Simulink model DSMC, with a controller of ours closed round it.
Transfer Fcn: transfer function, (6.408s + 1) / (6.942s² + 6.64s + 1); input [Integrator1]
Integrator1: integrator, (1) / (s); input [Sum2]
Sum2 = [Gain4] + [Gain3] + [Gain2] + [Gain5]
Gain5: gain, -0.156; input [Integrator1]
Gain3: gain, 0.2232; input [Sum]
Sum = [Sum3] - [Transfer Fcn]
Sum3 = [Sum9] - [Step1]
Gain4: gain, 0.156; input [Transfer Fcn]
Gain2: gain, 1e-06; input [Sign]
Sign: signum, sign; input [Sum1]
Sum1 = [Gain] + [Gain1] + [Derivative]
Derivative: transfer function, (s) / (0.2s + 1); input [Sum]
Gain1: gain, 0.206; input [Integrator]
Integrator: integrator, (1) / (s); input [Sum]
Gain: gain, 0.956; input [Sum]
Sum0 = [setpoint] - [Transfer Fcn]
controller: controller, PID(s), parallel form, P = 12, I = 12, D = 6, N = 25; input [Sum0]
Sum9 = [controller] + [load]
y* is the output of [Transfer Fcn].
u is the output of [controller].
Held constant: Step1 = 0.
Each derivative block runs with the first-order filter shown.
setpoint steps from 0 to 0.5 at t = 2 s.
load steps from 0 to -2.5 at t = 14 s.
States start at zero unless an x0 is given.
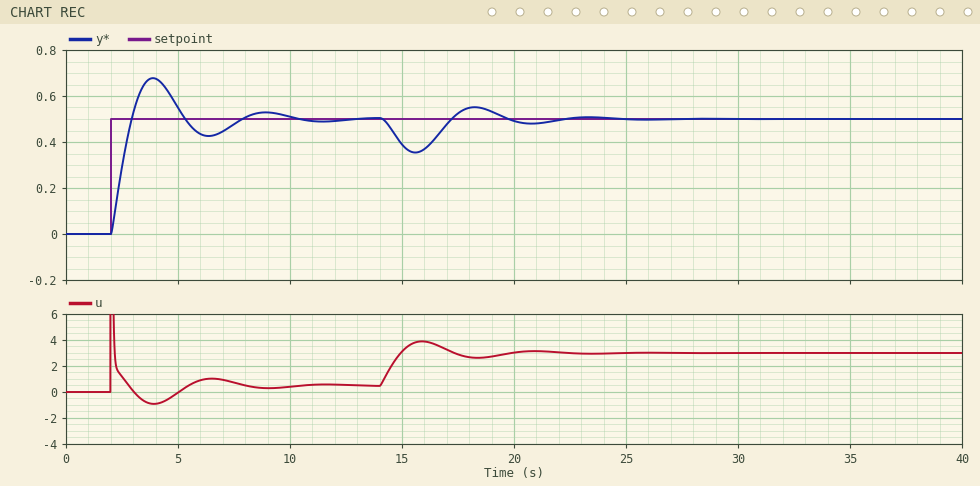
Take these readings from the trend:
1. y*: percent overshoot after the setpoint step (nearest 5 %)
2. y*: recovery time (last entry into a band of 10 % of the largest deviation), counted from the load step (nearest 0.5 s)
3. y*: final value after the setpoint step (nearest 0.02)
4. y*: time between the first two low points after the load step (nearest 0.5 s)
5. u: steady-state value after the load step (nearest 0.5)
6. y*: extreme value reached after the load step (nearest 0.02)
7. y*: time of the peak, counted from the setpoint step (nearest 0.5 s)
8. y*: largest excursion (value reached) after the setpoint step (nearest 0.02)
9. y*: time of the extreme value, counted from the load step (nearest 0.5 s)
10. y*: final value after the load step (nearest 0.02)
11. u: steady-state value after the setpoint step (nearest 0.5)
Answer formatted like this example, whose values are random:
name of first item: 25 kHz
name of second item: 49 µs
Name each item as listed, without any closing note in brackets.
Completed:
y*: percent overshoot after the setpoint step: 35 %
y*: recovery time (last entry into a band of 10 % of the largest deviation), counted from the load step: 7.5 s
y*: final value after the setpoint step: 0.50
y*: time between the first two low points after the load step: 5.0 s
u: steady-state value after the load step: 3.0
y*: extreme value reached after the load step: 0.36
y*: time of the peak, counted from the setpoint step: 2.0 s
y*: largest excursion (value reached) after the setpoint step: 0.68
y*: time of the extreme value, counted from the load step: 1.5 s
y*: final value after the load step: 0.50
u: steady-state value after the setpoint step: 0.5
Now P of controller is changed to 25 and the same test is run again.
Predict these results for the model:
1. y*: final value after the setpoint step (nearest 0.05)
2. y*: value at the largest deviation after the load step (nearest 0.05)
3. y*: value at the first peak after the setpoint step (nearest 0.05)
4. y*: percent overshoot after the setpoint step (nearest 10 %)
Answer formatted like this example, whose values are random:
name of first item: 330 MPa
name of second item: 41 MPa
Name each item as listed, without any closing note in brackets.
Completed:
y*: final value after the setpoint step: 0.50
y*: value at the largest deviation after the load step: 0.40
y*: value at the first peak after the setpoint step: 0.65
y*: percent overshoot after the setpoint step: 30 %
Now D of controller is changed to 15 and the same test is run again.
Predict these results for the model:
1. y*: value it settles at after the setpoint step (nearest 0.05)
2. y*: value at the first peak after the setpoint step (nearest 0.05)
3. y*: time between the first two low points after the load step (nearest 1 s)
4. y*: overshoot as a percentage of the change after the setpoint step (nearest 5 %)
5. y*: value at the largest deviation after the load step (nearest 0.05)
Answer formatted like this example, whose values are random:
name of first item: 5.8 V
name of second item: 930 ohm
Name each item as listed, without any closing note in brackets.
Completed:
y*: value it settles at after the setpoint step: 0.50
y*: value at the first peak after the setpoint step: 0.55
y*: time between the first two low points after the load step: 8 s
y*: overshoot as a percentage of the change after the setpoint step: 10 %
y*: value at the largest deviation after the load step: 0.40
